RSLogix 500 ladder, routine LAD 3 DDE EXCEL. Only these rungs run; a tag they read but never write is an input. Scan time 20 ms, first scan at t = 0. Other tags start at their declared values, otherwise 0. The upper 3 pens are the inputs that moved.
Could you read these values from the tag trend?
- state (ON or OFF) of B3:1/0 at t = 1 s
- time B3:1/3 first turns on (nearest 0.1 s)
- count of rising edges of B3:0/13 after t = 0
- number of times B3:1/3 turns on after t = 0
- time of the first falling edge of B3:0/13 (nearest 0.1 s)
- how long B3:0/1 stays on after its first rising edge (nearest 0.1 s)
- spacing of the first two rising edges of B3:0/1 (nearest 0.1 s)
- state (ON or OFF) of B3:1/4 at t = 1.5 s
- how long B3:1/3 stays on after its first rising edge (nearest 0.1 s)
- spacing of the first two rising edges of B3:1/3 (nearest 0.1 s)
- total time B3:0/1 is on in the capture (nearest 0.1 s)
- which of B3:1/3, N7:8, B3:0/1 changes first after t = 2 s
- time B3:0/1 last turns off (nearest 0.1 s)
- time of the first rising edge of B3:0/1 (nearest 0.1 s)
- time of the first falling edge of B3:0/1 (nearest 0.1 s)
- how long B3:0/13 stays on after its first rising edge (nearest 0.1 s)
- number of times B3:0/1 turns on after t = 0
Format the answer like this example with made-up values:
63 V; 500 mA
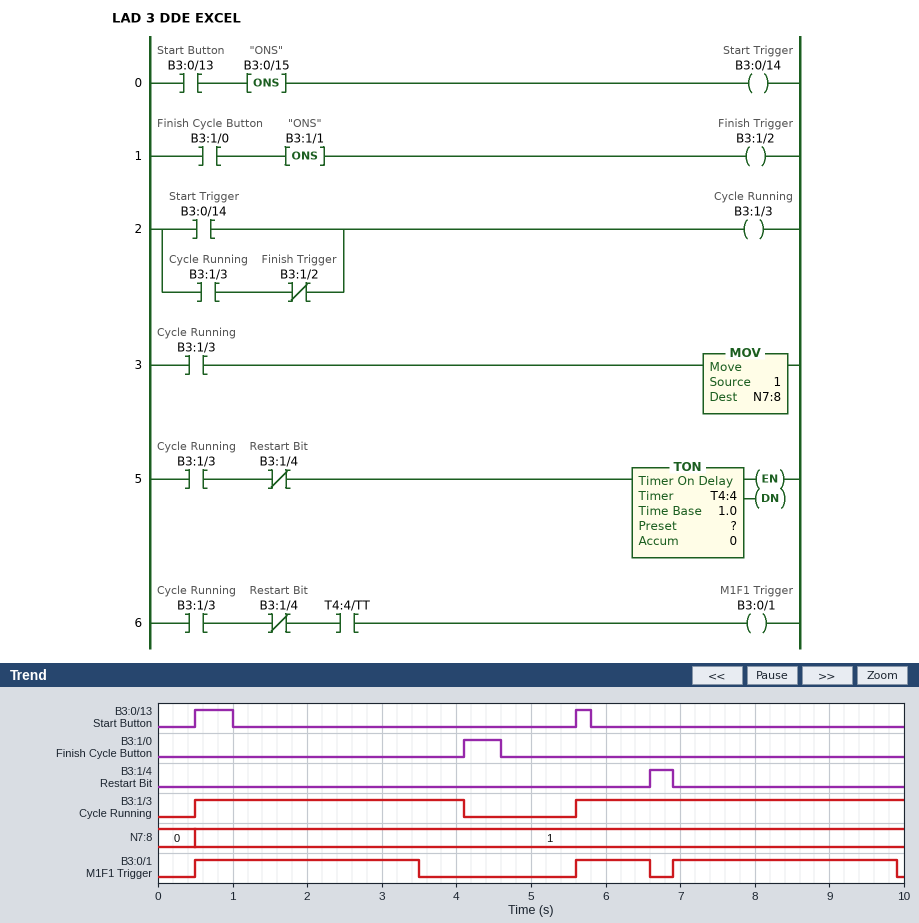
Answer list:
OFF; 0.5 s; 2; 2; 1.0 s; 3.0 s; 5.1 s; OFF; 3.6 s; 5.1 s; 7.0 s; B3:0/1; 9.9 s; 0.5 s; 3.5 s; 0.5 s; 3
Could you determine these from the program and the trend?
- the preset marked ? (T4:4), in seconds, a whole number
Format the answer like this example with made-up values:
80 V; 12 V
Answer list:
3 s
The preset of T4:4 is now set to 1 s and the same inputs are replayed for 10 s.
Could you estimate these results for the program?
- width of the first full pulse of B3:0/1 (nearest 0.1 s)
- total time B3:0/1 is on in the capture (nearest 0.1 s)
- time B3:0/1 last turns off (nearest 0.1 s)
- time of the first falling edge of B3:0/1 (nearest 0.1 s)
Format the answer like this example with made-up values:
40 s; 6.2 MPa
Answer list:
1.0 s; 3.0 s; 7.9 s; 1.5 s
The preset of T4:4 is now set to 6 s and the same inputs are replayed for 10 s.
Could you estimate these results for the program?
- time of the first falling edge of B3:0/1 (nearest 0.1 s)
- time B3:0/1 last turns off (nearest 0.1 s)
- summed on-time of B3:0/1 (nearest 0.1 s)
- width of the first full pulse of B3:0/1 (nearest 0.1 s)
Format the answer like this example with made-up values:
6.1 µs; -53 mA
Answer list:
4.1 s; 6.6 s; 7.7 s; 3.6 s
